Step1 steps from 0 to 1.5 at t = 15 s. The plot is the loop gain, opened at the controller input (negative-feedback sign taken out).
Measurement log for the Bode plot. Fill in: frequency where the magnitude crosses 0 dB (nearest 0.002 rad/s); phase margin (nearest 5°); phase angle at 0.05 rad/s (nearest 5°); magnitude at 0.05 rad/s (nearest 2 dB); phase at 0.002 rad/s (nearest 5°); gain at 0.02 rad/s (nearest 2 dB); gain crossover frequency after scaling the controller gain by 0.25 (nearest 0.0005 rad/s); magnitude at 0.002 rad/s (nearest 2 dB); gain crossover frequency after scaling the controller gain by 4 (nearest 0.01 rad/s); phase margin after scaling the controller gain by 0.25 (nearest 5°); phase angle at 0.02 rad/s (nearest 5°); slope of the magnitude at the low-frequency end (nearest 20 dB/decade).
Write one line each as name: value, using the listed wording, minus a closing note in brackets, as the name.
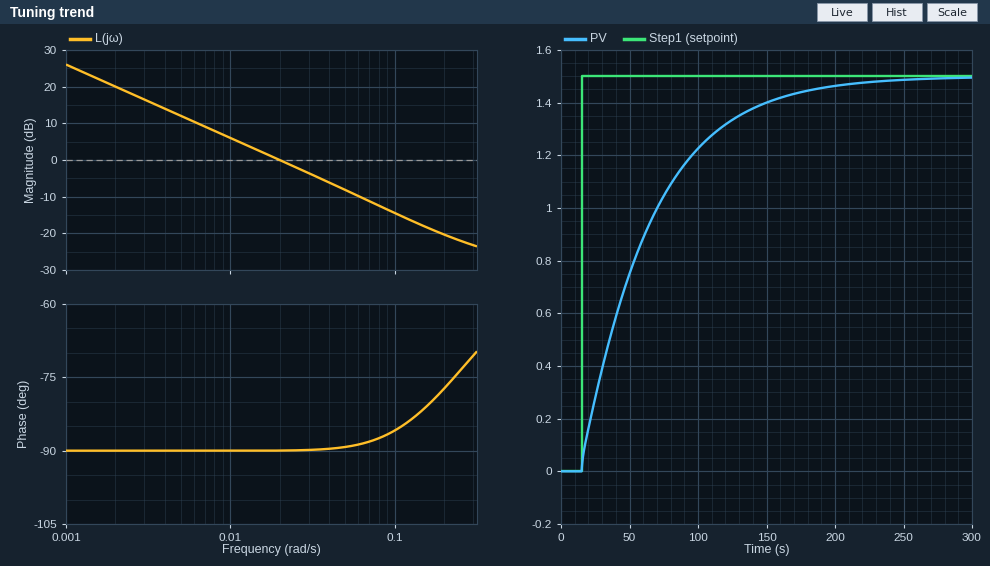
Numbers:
frequency where the magnitude crosses 0 dB: 0.020 rad/s
phase margin: 90°
phase angle at 0.05 rad/s: -90°
magnitude at 0.05 rad/s: -8 dB
phase at 0.002 rad/s: -90°
gain at 0.02 rad/s: 0 dB
gain crossover frequency after scaling the controller gain by 0.25: 0.0050 rad/s
magnitude at 0.002 rad/s: 20 dB
gain crossover frequency after scaling the controller gain by 4: 0.08 rad/s
phase margin after scaling the controller gain by 0.25: 90°
phase angle at 0.02 rad/s: -90°
slope of the magnitude at the low-frequency end: -20 dB/decade
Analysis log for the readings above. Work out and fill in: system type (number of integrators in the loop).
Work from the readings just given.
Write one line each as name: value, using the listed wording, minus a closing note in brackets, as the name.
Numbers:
system type: 1
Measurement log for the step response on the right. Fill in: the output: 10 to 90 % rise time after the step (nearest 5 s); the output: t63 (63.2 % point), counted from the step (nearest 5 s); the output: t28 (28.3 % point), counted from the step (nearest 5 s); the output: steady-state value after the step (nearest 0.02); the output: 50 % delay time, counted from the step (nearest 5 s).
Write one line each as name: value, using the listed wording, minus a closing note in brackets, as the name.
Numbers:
the output: 10 to 90 % rise time after the step: 110 s
the output: t63 (63.2 % point), counted from the step: 50 s
the output: t28 (28.3 % point), counted from the step: 15 s
the output: steady-state value after the step: 1.50
the output: 50 % delay time, counted from the step: 35 s
